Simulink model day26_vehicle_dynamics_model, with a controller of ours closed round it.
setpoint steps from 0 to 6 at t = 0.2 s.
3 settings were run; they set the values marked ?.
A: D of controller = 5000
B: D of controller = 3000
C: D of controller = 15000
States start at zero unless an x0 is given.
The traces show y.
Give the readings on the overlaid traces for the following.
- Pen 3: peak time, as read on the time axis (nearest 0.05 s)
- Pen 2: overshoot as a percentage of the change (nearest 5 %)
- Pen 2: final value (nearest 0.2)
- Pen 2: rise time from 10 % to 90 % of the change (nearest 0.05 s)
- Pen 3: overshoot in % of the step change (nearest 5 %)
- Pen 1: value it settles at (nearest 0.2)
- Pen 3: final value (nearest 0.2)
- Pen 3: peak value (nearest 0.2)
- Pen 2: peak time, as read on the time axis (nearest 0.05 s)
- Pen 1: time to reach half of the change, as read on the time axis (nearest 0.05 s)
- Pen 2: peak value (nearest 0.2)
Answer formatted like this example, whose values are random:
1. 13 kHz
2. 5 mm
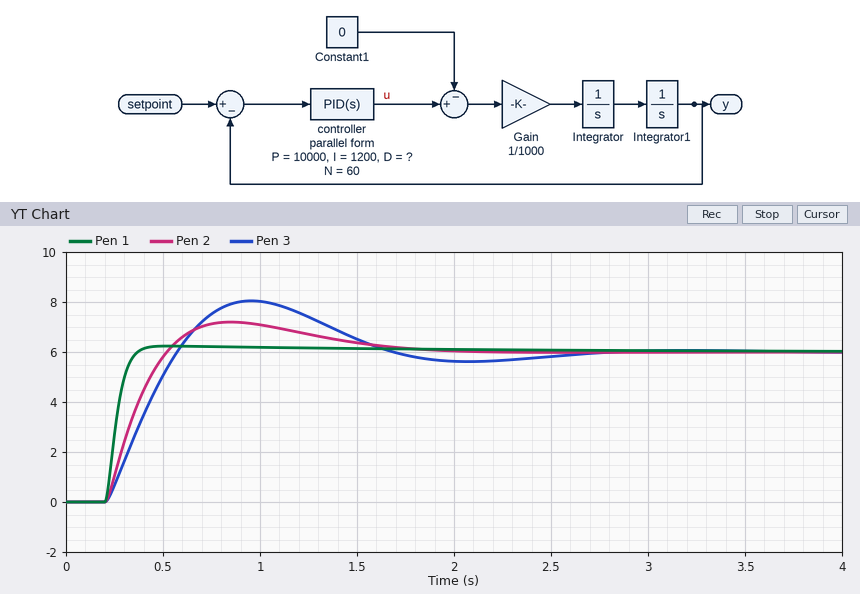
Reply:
1. 0.95 s
2. 20 %
3. 6.0
4. 0.25 s
5. 35 %
6. 6.0
7. 6.0
8. 8.0
9. 0.85 s
10. 0.25 s
11. 7.2
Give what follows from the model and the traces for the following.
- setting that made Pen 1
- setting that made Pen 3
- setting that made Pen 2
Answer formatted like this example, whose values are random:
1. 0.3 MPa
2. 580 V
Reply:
1. C
2. B
3. A
